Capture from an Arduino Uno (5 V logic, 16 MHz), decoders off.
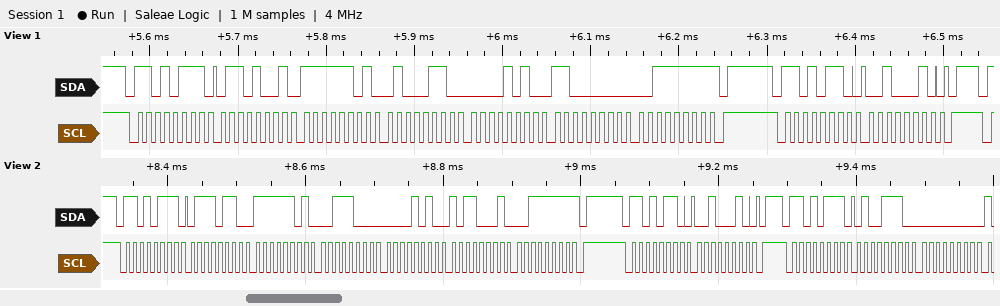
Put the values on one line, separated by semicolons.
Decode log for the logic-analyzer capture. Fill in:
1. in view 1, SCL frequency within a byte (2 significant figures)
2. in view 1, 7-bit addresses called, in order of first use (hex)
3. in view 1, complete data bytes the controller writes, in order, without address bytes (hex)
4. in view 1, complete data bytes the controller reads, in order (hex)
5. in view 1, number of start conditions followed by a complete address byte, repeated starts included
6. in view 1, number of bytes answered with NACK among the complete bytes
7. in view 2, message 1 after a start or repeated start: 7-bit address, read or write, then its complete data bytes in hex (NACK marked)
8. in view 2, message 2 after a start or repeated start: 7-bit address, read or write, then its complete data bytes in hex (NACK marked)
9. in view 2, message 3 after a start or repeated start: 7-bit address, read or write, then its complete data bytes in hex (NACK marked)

100 kHz; 0x6B; 22; 69 FD 46 0A C0 3F; 2; 1; 0x6B read: 76 FD 38 0A B1 3F NACK; 0x6B write: 22; 0x6B read: 4E 00
